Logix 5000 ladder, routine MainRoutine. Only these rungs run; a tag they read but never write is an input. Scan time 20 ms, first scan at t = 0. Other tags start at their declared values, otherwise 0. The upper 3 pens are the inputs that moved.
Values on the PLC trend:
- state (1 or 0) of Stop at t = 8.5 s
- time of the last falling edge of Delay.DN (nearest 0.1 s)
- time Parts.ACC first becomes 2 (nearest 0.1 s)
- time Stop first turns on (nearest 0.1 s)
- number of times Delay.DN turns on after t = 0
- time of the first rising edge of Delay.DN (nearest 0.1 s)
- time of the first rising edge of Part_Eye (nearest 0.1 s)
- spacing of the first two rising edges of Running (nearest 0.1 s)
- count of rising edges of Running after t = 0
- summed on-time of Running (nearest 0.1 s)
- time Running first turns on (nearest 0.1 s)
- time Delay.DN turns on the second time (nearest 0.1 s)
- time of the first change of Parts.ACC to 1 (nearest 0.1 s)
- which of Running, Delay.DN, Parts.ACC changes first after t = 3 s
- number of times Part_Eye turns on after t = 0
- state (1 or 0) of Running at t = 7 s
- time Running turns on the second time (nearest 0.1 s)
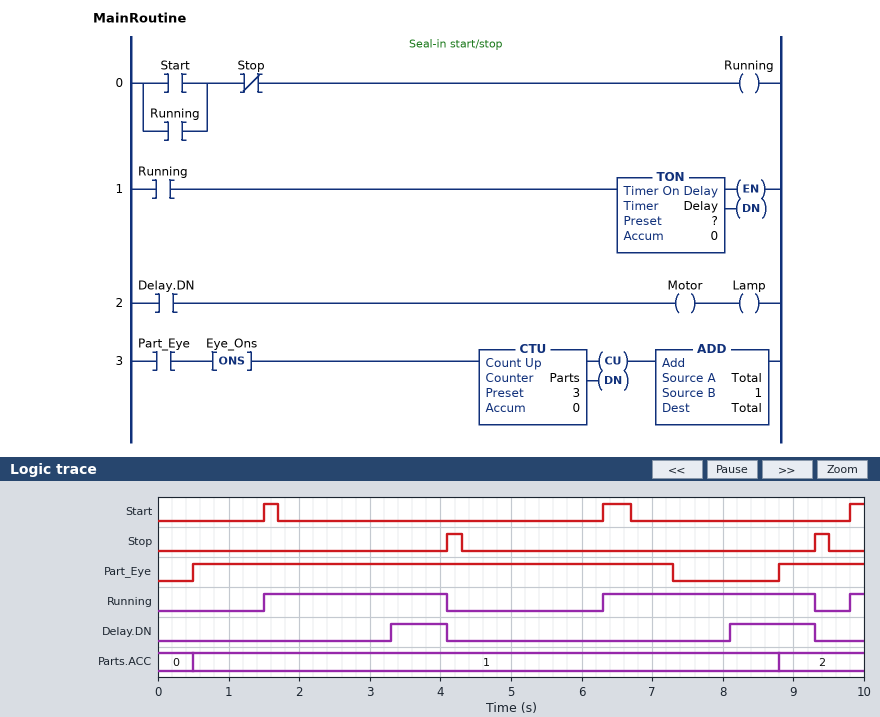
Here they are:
0
9.3 s
8.8 s
4.1 s
2
3.3 s
0.5 s
4.8 s
3
5.8 s
1.5 s
8.1 s
0.5 s
Delay.DN
2
1
6.3 s
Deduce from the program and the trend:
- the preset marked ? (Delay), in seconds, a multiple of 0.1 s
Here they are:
1.8 s
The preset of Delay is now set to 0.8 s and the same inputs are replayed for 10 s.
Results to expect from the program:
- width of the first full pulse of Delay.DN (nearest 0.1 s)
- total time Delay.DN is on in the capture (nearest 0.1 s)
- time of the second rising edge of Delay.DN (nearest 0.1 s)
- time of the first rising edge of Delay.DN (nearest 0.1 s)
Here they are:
1.8 s
4.0 s
7.1 s
2.3 s
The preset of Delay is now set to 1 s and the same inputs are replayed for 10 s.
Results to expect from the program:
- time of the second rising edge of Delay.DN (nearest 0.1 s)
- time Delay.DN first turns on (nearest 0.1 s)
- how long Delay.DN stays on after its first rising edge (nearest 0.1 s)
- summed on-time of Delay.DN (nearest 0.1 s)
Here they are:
7.3 s
2.5 s
1.6 s
3.6 s
